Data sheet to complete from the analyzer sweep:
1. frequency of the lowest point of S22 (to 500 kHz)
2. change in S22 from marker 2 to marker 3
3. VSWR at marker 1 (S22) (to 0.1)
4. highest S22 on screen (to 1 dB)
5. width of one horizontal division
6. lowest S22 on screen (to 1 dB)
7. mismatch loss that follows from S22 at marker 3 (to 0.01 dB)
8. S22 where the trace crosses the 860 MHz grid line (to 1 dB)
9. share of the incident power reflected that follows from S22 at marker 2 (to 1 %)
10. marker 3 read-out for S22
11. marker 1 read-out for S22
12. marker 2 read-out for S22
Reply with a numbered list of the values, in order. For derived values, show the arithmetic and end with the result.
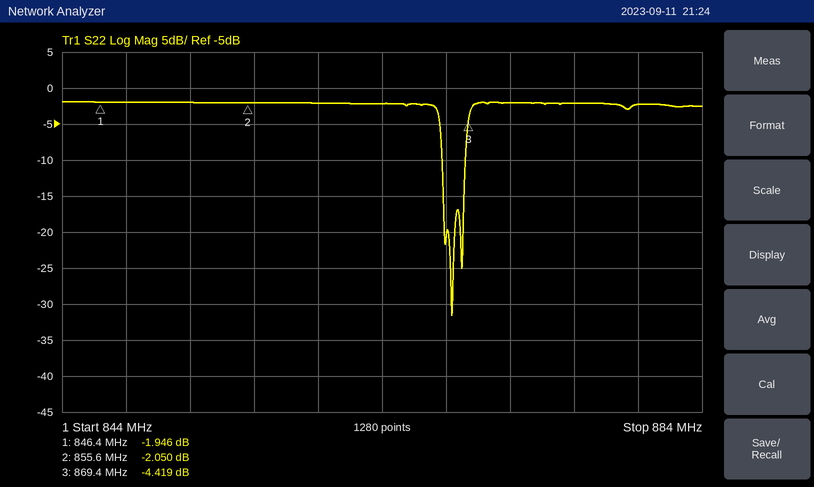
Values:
1. 868.5 MHz
2. -4.419 − (-2.05) = -2.369 dB
3. (1 + 0.7993)/(1 − 0.7993) ≈ 9.0
4. -2 dB
5. 4 MHz
6. -32 dB
7. −10 log10(1 − 10^(-4.419/10)) ≈ 1.95 dB
8. -2 dB
9. 10^(-2.05/10) ≈ 62 %
10. -4.419 dB
11. -1.946 dB
12. -2.050 dB
